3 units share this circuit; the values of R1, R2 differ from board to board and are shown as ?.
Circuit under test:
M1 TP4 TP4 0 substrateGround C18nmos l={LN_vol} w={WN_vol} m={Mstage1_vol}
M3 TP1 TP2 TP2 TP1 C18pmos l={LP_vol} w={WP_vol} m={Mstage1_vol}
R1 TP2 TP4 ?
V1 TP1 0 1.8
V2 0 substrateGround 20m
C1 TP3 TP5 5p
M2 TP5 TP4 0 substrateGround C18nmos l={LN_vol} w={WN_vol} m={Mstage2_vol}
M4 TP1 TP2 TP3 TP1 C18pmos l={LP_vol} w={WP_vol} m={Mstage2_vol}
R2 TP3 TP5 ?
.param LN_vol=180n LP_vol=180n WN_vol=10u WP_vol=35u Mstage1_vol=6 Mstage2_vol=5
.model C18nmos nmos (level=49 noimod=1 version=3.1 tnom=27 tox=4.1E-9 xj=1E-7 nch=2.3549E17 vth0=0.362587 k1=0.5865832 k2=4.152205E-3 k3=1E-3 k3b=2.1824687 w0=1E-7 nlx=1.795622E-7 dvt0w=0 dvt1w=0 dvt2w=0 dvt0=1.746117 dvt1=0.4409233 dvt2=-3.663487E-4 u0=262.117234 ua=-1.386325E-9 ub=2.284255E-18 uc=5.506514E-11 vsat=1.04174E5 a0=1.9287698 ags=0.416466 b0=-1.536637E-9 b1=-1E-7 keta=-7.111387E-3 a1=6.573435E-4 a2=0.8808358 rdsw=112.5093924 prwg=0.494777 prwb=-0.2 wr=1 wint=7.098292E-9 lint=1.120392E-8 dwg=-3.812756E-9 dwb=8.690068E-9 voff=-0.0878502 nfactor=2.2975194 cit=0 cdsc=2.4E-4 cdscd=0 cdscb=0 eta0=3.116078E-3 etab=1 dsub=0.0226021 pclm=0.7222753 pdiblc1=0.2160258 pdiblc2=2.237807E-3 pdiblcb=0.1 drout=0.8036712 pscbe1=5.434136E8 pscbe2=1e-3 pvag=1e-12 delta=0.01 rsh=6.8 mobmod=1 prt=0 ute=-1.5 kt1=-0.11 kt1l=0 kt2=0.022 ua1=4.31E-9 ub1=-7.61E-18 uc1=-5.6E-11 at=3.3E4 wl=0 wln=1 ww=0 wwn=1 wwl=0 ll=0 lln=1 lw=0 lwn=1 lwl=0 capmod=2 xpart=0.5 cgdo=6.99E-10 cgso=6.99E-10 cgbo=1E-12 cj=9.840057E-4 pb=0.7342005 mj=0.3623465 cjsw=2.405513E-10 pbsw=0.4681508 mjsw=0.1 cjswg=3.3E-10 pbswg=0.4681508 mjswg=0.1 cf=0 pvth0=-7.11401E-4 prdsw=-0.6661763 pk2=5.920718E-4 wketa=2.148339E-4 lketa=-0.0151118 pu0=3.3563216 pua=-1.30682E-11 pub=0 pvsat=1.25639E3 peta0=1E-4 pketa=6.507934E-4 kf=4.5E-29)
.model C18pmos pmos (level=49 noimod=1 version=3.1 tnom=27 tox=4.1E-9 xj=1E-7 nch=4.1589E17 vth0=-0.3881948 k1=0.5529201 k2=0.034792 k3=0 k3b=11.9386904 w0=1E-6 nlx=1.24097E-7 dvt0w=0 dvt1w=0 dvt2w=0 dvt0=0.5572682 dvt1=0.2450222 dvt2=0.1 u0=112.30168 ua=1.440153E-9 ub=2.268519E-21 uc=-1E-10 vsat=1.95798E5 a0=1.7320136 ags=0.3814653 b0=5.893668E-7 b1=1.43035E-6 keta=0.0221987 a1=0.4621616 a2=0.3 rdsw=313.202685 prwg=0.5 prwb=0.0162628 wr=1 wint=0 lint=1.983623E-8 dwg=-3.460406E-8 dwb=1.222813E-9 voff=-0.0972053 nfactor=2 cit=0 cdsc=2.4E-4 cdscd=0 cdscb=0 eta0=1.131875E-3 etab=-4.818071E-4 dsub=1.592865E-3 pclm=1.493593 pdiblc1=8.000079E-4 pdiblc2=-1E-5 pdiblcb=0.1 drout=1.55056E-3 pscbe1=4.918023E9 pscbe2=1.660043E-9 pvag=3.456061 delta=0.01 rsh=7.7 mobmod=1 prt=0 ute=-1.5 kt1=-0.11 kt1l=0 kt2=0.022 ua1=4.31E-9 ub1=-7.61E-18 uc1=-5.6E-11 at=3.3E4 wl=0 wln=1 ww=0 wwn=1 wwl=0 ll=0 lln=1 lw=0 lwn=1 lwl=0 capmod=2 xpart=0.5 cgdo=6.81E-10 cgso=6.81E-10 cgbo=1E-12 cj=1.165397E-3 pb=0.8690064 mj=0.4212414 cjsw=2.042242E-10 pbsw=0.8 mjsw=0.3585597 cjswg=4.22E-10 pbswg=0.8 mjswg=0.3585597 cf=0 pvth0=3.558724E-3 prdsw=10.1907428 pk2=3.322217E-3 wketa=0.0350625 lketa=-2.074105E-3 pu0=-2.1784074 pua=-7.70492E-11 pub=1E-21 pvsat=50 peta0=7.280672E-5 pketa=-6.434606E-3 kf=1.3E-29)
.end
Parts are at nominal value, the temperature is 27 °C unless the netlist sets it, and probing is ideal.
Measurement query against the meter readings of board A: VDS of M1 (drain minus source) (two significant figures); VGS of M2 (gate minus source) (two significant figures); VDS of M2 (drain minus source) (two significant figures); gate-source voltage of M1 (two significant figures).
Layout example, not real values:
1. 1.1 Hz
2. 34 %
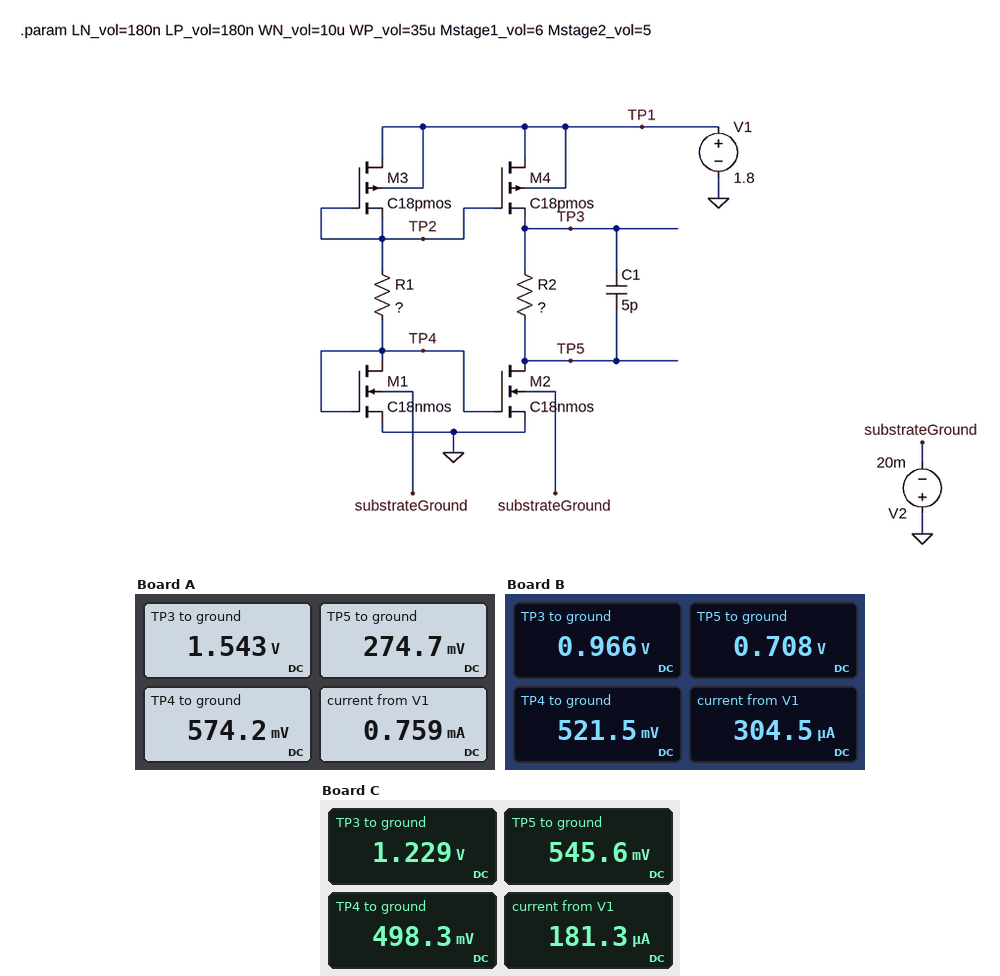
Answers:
1. 570 mV
2. 570 mV
3. 270 mV
4. 570 mV
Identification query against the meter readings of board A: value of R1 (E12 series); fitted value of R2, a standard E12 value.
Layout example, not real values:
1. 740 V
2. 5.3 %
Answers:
1. 1.5 kΩ
2. 3.9 kΩ
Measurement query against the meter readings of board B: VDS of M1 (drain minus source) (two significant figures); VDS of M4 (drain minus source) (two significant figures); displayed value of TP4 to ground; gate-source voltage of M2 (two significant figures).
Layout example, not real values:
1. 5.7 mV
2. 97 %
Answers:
1. 520 mV
2. 830 mV
3. 521.5 mV
4. 520 mV
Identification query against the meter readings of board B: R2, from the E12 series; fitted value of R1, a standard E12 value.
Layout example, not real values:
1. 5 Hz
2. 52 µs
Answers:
1. 1.8 kΩ
2. 4.7 kΩ
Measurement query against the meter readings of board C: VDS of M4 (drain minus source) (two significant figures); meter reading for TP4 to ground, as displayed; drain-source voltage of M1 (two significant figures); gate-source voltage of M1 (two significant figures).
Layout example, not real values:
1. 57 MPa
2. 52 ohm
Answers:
1. 570 mV
2. 498.3 mV
3. 500 mV
4. 500 mV
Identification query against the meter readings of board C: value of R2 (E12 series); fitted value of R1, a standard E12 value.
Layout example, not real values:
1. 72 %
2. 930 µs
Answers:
1. 8.2 kΩ
2. 8.2 kΩ
